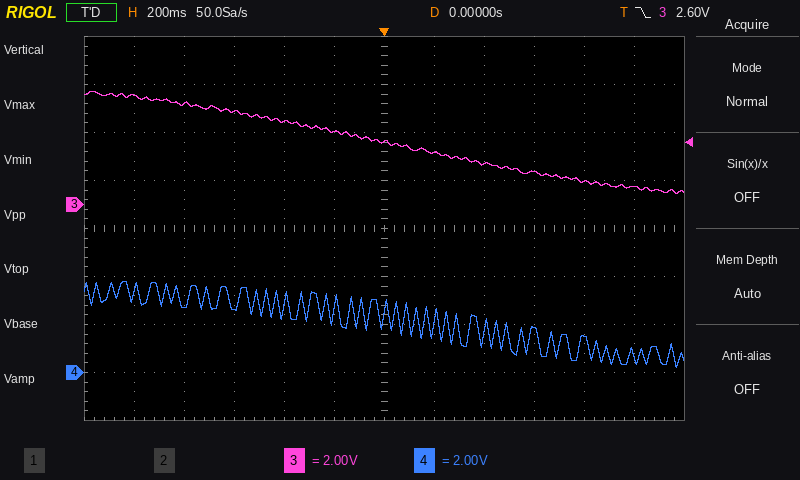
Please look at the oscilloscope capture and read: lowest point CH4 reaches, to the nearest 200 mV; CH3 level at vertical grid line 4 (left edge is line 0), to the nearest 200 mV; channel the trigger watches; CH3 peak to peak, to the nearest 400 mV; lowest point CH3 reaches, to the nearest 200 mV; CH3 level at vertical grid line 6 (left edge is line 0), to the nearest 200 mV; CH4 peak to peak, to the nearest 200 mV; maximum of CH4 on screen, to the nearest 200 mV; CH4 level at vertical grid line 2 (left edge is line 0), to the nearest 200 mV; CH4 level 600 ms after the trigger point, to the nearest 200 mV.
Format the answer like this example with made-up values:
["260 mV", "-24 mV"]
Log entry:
["200 mV", "3.4 V", "CH3", "4.4 V", "400 mV", "2.6 V", "3.6 V", "3.8 V", "2.8 V", "1.8 V"]
